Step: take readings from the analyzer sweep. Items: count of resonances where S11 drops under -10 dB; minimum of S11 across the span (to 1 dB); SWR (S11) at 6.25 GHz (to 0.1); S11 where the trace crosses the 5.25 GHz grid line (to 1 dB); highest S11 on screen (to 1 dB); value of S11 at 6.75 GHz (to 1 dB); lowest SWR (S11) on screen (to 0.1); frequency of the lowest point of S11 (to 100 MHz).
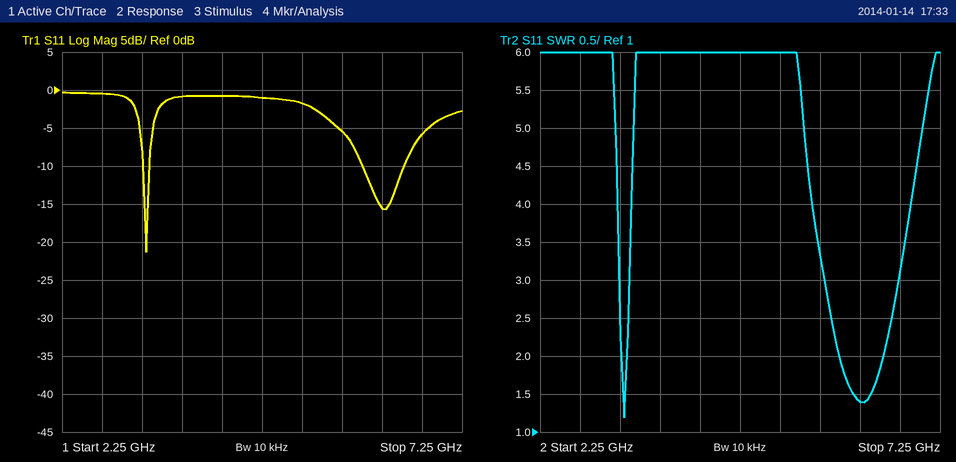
2
-21 dB
1.4
-2 dB
0 dB
-6 dB
1.2
3.3 GHz
